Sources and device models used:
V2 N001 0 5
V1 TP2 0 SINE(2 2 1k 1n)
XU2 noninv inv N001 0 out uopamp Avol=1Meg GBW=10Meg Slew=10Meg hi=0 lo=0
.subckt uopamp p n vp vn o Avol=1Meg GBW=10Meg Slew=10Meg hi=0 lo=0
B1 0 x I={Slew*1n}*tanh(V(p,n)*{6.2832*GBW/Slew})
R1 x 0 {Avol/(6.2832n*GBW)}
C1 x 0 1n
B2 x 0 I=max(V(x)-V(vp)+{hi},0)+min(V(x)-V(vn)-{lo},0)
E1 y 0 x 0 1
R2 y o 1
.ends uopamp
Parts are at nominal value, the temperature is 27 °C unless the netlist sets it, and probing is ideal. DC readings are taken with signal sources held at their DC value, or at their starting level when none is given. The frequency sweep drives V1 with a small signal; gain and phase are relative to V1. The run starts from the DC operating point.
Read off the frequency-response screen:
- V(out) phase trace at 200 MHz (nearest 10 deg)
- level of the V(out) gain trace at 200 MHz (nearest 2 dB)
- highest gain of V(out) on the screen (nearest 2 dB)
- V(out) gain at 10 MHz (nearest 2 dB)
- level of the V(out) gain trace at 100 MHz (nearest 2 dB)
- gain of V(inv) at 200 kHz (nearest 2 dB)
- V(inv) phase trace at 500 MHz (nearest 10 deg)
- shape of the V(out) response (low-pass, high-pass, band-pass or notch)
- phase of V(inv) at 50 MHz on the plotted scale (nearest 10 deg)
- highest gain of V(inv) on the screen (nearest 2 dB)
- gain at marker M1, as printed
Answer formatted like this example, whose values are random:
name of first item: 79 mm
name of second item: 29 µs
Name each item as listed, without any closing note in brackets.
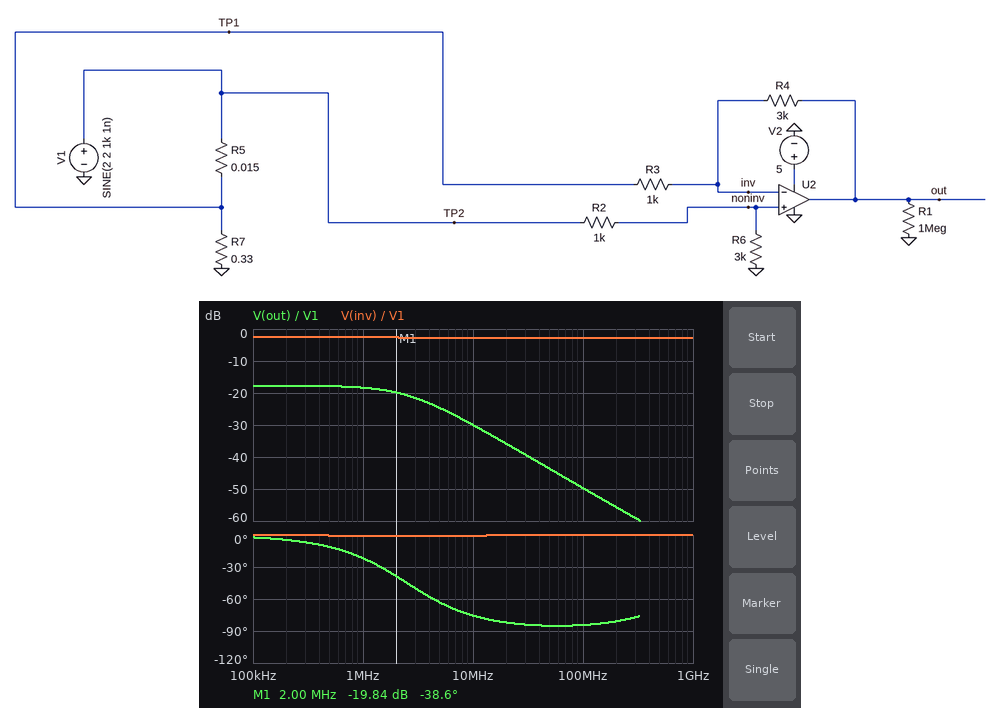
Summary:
V(out) phase trace at 200 MHz: -80 deg
level of the V(out) gain trace at 200 MHz: -56 dB
highest gain of V(out) on the screen: -18 dB
V(out) gain at 10 MHz: -30 dB
level of the V(out) gain trace at 100 MHz: -50 dB
gain of V(inv) at 200 kHz: -2 dB
V(inv) phase trace at 500 MHz: 0 deg
shape of the V(out) response: low-pass
phase of V(inv) at 50 MHz on the plotted scale: 0 deg
highest gain of V(inv) on the screen: -2 dB
gain at marker M1, as printed: -19.84 dB
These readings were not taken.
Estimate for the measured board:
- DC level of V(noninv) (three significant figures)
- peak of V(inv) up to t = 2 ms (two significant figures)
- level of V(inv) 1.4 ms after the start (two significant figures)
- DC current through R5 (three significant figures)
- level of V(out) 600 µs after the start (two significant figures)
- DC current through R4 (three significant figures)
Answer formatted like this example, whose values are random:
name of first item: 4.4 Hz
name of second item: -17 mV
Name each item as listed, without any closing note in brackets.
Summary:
DC level of V(noninv): 1.50 V
peak of V(inv) up to t = 2 ms: 3.0 V
level of V(inv) 1.4 ms after the start: 2.4 V
DC current through R5: 5.80 A
level of V(out) 600 µs after the start: 110 mV
DC current through R4: 413 µA
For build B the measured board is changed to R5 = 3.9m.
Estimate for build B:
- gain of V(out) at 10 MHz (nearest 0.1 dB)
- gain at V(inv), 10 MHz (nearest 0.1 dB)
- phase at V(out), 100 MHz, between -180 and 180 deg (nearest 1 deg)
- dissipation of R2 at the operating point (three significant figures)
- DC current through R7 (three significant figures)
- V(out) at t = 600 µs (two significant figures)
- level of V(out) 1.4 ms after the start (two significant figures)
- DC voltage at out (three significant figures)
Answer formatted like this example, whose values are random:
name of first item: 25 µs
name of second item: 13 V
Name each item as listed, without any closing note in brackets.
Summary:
gain of V(out) at 10 MHz: -41.4 dB
gain at V(inv), 10 MHz: -2.6 dB
phase at V(out), 100 MHz, between -180 and 180 deg: -73 deg
dissipation of R2 at the operating point: 250 µW
DC current through R7: 5.99 A
V(out) at t = 600 µs: 29 mV
level of V(out) 1.4 ms after the start: 110 mV
DC voltage at out: 70.1 mV
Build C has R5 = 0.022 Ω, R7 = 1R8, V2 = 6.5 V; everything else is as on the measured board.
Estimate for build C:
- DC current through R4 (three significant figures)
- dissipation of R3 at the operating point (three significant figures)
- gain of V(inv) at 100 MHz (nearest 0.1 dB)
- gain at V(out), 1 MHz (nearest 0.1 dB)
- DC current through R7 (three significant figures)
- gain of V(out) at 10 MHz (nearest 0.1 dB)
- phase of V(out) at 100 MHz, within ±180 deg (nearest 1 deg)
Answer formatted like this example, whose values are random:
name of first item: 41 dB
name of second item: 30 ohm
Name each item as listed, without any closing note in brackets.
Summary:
DC current through R4: 476 µA
dissipation of R3 at the operating point: 226 µW
gain of V(inv) at 100 MHz: -2.6 dB
gain at V(out), 1 MHz: -29.5 dB
DC current through R7: 1.10 A
gain of V(out) at 10 MHz: -41.1 dB
phase of V(out) at 100 MHz, within ±180 deg: -73 deg
